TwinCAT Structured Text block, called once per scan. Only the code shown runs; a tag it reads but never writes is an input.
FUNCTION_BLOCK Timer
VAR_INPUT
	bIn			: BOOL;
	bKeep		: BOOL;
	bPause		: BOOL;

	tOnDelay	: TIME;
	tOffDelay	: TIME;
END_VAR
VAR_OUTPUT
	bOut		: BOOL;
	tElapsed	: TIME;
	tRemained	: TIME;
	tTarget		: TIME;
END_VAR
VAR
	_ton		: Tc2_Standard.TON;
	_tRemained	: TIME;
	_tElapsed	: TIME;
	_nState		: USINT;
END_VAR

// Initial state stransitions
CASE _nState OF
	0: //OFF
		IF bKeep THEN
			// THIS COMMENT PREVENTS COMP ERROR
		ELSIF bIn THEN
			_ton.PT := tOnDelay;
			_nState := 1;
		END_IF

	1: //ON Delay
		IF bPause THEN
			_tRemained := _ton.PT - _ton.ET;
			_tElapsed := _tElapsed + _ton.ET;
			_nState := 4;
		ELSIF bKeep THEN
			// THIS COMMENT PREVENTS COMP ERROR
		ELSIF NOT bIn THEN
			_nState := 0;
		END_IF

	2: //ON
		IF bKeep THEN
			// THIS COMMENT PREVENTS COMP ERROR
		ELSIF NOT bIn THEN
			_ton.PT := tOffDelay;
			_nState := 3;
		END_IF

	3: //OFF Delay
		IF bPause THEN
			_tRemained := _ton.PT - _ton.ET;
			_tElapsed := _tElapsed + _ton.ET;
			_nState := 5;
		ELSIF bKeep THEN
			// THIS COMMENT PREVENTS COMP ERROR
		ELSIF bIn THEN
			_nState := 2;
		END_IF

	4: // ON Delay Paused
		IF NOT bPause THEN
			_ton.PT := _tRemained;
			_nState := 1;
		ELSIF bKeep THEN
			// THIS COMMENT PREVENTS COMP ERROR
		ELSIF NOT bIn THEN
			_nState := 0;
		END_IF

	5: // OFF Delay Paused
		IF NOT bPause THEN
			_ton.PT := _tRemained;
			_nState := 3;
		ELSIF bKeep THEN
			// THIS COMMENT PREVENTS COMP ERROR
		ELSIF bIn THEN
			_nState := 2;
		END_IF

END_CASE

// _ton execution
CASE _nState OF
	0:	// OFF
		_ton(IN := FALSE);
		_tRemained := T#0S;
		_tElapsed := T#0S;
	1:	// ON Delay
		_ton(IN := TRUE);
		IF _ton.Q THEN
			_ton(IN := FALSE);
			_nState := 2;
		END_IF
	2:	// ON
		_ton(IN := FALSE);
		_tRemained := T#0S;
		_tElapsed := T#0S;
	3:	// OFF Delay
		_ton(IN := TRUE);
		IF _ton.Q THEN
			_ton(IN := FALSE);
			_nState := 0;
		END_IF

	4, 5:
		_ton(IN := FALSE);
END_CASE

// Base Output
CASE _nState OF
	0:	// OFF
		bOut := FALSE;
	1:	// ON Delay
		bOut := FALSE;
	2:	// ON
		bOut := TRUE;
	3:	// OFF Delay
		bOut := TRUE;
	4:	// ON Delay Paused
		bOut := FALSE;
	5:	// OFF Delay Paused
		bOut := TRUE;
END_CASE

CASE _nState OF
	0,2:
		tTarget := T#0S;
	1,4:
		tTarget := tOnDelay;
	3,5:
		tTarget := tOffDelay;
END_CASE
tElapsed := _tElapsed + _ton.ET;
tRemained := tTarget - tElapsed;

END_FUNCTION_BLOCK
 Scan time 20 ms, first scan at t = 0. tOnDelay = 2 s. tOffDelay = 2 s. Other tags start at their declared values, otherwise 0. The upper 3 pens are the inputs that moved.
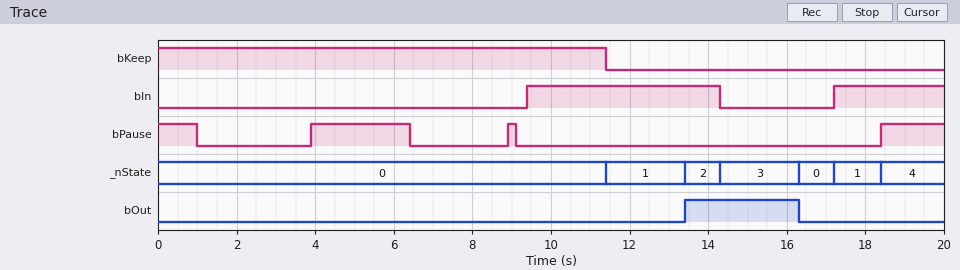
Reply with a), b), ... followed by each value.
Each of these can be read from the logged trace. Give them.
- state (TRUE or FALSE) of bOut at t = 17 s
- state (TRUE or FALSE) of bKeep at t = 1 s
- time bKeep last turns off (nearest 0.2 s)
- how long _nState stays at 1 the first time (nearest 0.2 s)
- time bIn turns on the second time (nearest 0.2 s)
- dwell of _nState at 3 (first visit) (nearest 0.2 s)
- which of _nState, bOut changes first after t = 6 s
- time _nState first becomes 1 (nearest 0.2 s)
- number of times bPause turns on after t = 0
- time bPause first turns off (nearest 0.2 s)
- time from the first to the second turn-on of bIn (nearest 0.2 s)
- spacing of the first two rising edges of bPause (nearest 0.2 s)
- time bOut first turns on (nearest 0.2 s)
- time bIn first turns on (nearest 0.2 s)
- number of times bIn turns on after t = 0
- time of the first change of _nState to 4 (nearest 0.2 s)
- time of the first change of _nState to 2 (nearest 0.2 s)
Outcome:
a) FALSE
b) TRUE
c) 11.4 s
d) 2.0 s
e) 17.2 s
f) 2.0 s
g) _nState
h) 11.4 s
i) 3
j) 1.0 s
k) 7.8 s
l) 5.0 s
m) 13.4 s
n) 9.4 s
o) 2
p) 18.4 s
q) 13.4 s
